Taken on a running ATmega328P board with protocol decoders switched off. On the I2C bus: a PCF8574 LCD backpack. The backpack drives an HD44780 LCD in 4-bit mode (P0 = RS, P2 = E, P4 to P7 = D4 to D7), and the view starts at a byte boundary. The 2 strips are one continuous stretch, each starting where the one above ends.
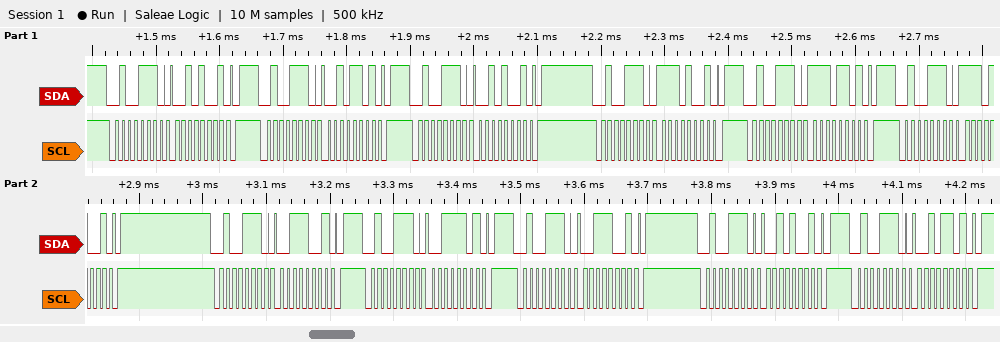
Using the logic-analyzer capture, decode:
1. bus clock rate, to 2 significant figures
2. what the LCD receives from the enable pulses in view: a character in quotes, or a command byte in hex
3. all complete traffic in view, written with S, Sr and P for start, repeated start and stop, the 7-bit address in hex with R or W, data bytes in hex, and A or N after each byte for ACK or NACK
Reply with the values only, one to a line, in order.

100 kHz
'.'
S 27W A 29 A P S 27W A 2D A P S 27W A 29 A P S 27W A E9 A P S 27W A ED A P S 27W A E9 A P S 27W A 39 A P S 27W A 3D A P S 27W A 39 A P S 27W A 29 A P S 27W A 2D A P
